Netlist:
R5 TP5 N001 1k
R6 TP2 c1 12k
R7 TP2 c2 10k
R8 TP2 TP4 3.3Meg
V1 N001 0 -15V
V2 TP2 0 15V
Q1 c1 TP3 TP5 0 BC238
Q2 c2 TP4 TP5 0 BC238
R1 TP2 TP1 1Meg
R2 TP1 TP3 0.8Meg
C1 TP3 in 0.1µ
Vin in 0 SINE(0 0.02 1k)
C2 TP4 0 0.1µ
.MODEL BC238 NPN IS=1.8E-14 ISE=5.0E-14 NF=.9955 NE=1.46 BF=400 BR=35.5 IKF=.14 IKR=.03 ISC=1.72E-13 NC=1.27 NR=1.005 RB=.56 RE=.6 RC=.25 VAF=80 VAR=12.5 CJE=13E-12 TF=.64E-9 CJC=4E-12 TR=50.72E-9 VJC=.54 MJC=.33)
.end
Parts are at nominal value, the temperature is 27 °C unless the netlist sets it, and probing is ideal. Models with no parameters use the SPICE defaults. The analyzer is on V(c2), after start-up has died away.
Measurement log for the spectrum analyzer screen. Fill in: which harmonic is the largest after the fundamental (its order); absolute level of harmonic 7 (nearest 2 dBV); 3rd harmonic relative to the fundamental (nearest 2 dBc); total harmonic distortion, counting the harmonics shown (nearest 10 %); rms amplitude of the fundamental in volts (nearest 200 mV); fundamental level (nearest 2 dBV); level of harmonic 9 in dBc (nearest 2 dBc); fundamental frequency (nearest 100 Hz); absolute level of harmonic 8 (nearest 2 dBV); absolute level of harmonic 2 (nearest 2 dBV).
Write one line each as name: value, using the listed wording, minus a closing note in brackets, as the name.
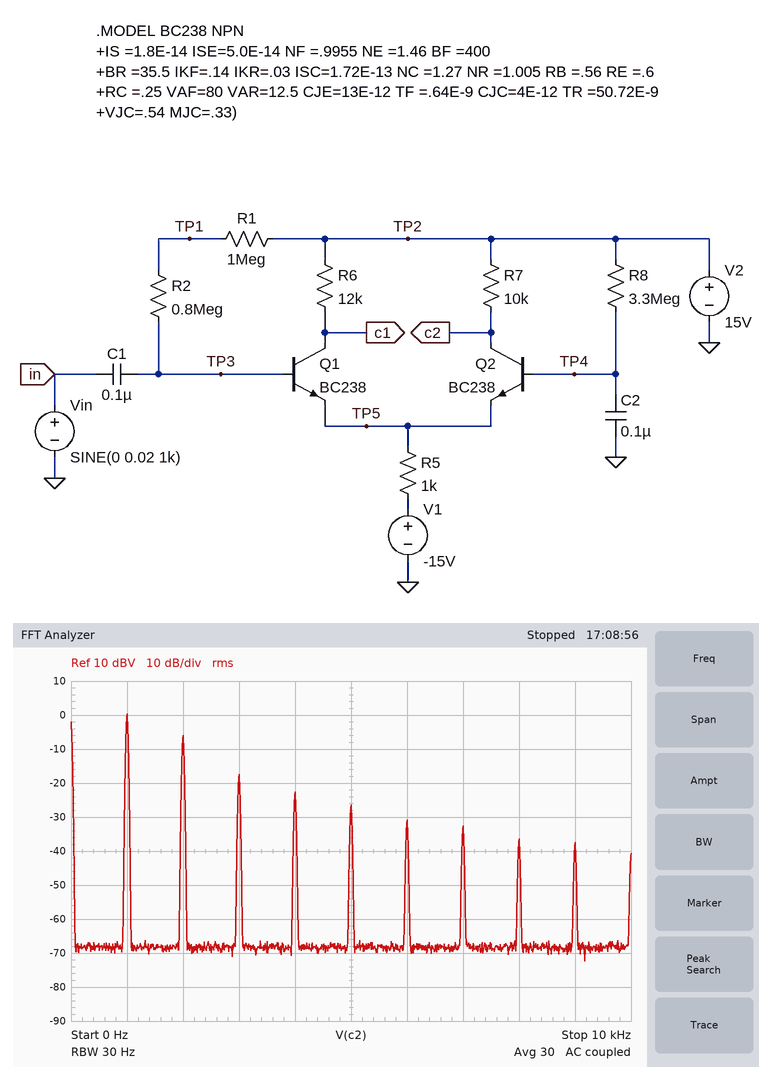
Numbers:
which harmonic is the largest after the fundamental: 2
absolute level of harmonic 7: -32 dBV
3rd harmonic relative to the fundamental: -18 dBc
total harmonic distortion, counting the harmonics shown: 50 %
rms amplitude of the fundamental in volts: 1.0 V
fundamental level: 0 dBV
level of harmonic 9 in dBc: -38 dBc
fundamental frequency: 1.0 kHz
absolute level of harmonic 8: -36 dBV
absolute level of harmonic 2: -6 dBV
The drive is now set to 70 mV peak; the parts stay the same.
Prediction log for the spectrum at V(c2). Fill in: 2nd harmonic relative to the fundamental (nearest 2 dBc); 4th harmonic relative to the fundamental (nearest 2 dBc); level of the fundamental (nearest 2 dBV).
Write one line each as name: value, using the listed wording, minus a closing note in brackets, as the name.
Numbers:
2nd harmonic relative to the fundamental: -18 dBc
4th harmonic relative to the fundamental: -28 dBc
level of the fundamental: 16 dBV
